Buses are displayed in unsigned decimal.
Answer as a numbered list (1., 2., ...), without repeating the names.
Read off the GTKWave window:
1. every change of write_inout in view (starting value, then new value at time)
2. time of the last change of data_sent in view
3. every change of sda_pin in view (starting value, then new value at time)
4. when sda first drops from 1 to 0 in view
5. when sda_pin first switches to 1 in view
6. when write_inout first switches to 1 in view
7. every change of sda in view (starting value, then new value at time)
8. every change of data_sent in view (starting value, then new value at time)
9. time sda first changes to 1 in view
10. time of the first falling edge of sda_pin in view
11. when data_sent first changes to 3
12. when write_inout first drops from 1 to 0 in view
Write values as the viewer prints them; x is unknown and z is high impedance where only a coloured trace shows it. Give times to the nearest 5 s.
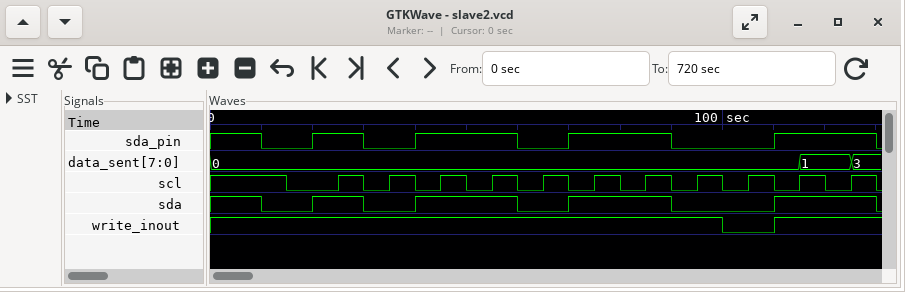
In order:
1. 1, 0 at 100 s, 1 at 110 s
2. 125 s
3. 1, 0 at 10 s, 1 at 20 s, 0 at 30 s, 1 at 40 s, 0 at 60 s, 1 at 70 s, 0 at 90 s, 1 at 110 s, 0 at 130 s
4. 10 s
5. 20 s
6. 110 s
7. 1, 0 at 10 s, 1 at 20 s, 0 at 30 s, 1 at 40 s, 0 at 60 s, 1 at 70 s, 0 at 90 s, 1 at 110 s, 0 at 130 s
8. 0, 1 at 115 s, 3 at 125 s
9. 20 s
10. 10 s
11. 125 s
12. 100 s
